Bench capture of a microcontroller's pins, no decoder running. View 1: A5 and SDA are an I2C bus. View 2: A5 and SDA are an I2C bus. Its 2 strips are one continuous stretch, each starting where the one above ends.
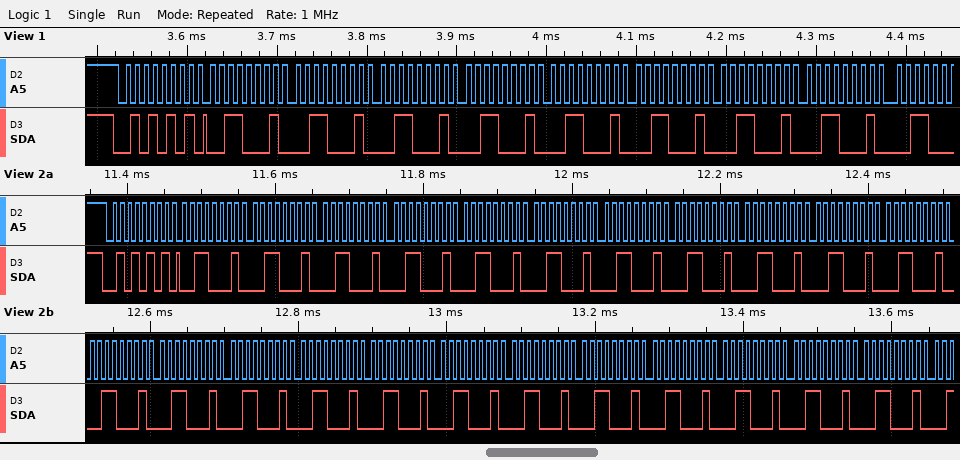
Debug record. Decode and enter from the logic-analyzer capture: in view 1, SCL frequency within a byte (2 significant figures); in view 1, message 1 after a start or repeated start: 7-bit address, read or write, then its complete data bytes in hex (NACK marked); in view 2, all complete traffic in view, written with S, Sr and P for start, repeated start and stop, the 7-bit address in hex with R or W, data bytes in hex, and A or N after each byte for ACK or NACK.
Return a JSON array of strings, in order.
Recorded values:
["100 kHz", "0x2A read: 31 31 31 31 31 31 31 31", "S 2AR A 31 A 31 A 31 A 31 A 31 A 31 A 31 A 31 A 31 A 31 A 31 A 31 A 31 A 31 A 31 A 31 A 31 A 31 A 31 A 31 A 31 A 31 A 31 A"]
